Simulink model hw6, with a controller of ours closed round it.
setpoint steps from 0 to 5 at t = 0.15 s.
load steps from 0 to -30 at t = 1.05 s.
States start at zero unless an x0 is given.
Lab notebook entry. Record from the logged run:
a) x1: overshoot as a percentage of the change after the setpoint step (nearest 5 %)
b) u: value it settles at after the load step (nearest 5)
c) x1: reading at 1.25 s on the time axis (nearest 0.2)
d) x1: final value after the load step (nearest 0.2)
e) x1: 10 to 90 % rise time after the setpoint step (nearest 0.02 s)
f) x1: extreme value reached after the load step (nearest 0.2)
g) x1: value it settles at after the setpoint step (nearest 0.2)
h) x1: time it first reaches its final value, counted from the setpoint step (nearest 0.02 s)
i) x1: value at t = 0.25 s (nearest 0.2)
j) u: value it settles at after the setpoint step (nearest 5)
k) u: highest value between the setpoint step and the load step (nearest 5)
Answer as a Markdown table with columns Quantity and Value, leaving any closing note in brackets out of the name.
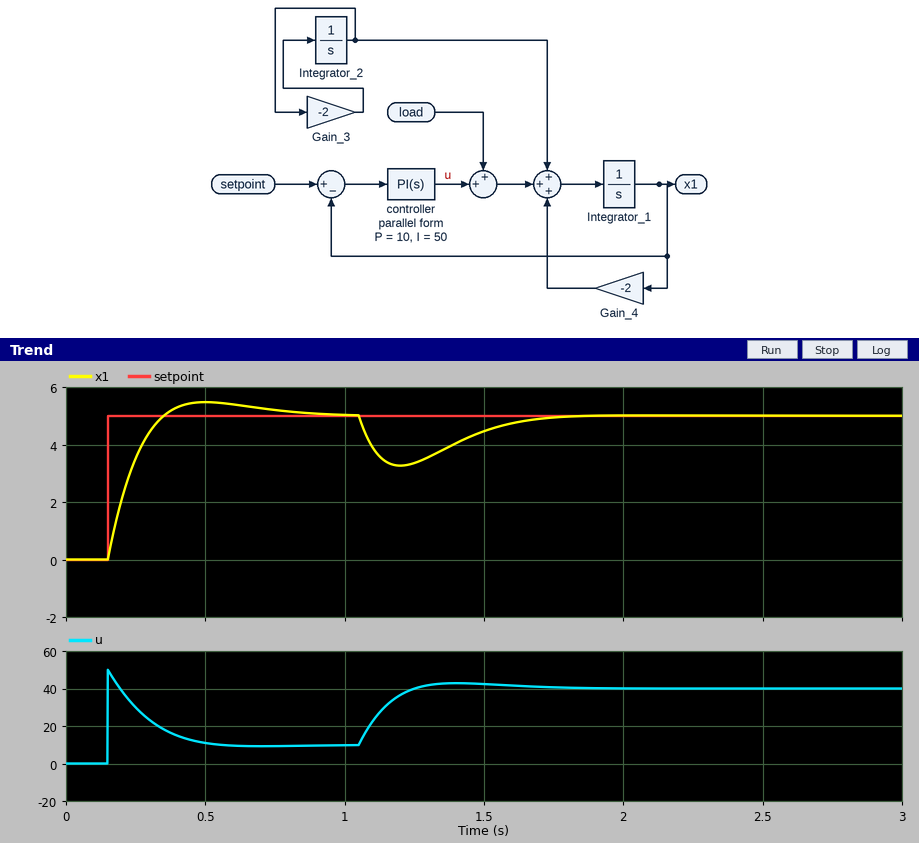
| Quantity | Value |
|---|---|
| x1: overshoot as a percentage of the change after the setpoint step | 10 % |
| u: value it settles at after the load step | 40 |
| x1: reading at 1.25 s on the time axis | 3.4 |
| x1: final value after the load step | 5.0 |
| x1: 10 to 90 % rise time after the setpoint step | 0.14 s |
| x1: extreme value reached after the load step | 3.2 |
| x1: value it settles at after the setpoint step | 5.0 |
| x1: time it first reaches its final value, counted from the setpoint step | 0.20 s |
| x1: value at t = 0.25 s | 3.6 |
| u: value it settles at after the setpoint step | 10 |
| u: highest value between the setpoint step and the load step | 50 |
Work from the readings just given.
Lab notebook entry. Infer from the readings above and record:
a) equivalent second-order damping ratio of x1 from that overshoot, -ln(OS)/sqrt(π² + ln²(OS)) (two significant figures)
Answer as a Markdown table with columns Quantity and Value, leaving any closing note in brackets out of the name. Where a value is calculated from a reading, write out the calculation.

| Quantity | Value |
|---|---|
| equivalent second-order damping ratio of x1 from that overshoot, -ln(OS)/sqrt(π² + ln²(OS)) | ln(0.1) = -2.303; 2.303 / sqrt(9.870 + 5.302) = 0.59 |
